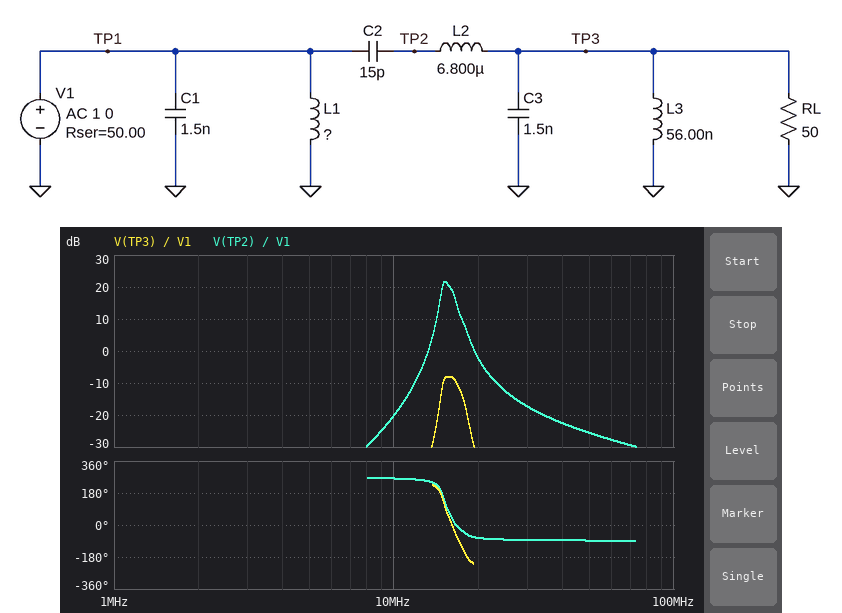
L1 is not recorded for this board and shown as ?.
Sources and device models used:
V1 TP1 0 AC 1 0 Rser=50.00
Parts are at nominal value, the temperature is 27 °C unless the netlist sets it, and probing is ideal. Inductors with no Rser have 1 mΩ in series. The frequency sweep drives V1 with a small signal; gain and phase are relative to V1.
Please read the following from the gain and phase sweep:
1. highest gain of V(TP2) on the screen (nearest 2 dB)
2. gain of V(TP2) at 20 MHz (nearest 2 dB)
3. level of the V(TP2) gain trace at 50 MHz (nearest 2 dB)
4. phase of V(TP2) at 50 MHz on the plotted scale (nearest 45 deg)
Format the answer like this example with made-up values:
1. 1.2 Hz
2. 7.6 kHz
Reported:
1. 22 dB
2. -2 dB
3. -26 dB
4. -90 deg
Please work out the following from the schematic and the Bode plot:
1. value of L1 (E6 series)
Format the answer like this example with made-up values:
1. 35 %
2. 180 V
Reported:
1. 68 nH
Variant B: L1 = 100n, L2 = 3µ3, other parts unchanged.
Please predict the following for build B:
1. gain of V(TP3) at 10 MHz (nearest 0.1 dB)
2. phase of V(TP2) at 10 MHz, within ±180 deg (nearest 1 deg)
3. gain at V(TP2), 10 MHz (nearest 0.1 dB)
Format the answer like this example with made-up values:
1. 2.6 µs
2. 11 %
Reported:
1. -54.7 dB
2. -108 deg
3. -22.5 dB
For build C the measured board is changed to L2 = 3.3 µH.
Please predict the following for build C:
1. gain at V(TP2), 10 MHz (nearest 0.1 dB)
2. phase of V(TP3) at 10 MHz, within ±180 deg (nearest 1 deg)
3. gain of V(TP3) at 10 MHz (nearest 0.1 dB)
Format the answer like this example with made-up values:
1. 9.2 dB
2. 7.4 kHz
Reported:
1. -28.9 dB
2. -104 deg
3. -61.1 dB
